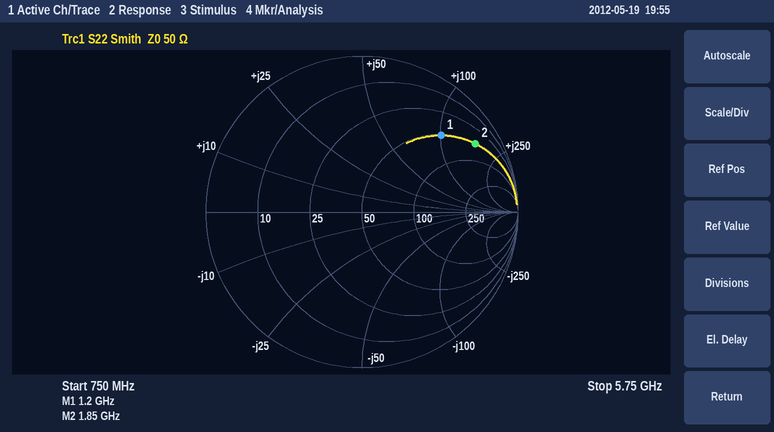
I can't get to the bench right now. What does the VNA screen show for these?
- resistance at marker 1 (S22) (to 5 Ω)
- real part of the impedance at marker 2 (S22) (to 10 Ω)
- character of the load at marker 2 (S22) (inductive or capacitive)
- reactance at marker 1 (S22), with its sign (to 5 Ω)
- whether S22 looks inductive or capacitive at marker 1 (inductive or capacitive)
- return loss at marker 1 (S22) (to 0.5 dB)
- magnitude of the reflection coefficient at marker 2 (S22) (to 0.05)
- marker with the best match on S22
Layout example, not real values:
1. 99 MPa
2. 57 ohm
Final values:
1. 50 Ω
2. 50 Ω
3. inductive
4. +100 Ω
5. inductive
6. 3.0 dB
7. 0.85
8. marker 1
